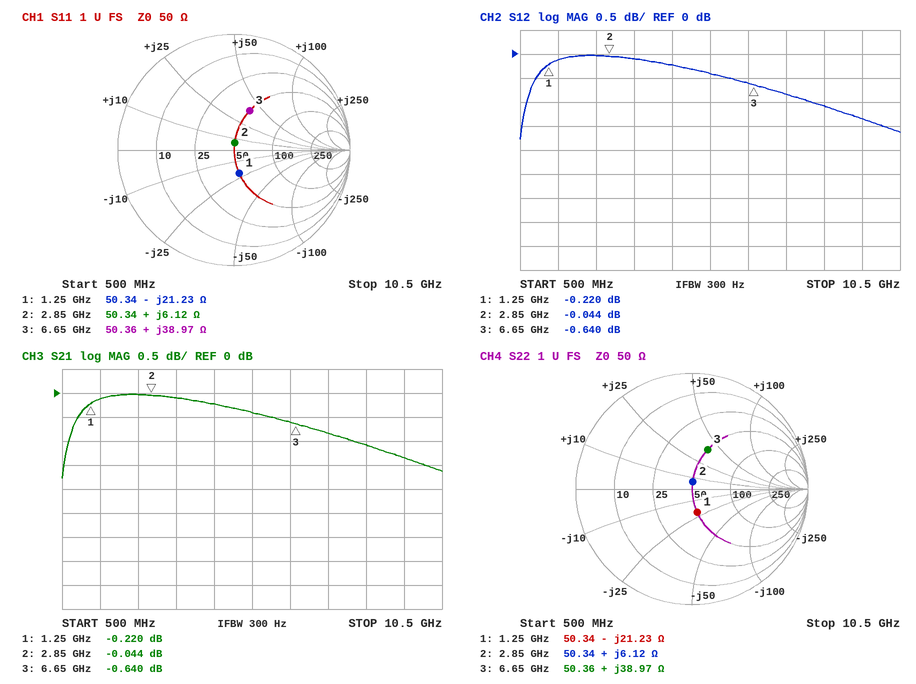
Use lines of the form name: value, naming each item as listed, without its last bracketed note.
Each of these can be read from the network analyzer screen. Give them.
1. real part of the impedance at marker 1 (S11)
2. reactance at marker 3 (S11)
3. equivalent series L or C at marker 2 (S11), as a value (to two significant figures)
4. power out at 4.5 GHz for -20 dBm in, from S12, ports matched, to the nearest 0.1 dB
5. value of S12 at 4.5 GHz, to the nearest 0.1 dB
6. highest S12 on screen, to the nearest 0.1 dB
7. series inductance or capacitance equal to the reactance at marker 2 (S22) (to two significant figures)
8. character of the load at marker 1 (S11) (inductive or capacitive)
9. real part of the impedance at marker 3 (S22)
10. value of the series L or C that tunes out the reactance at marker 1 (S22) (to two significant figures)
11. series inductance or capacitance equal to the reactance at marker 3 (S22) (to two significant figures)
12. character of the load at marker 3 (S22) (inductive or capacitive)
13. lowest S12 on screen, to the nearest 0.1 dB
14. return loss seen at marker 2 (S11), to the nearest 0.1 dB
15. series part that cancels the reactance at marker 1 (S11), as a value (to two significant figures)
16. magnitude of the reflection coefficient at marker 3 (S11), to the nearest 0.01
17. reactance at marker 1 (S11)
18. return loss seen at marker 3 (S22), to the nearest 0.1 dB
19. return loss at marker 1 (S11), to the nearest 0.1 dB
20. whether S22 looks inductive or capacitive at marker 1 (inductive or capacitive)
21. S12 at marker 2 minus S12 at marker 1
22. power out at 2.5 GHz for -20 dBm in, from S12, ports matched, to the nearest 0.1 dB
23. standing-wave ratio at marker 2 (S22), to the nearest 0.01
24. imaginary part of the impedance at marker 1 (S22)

real part of the impedance at marker 1: 50.34 Ω
reactance at marker 3: +38.97 Ω
equivalent series L or C at marker 2 (S11), as a value: 340 pH
power out at 4.5 GHz for -20 dBm in, from S12, ports matched, to the nearest 0.1 dB: -20.2 dBm
value of S12 at 4.5 GHz, to the nearest 0.1 dB: -0.2 dB
highest S12 on screen, to the nearest 0.1 dB: 0.0 dB
series inductance or capacitance equal to the reactance at marker 2 (S22): 340 pH
character of the load at marker 1 (S11): capacitive
real part of the impedance at marker 3: 50.36 Ω
value of the series L or C that tunes out the reactance at marker 1 (S22): 2.7 nH
series inductance or capacitance equal to the reactance at marker 3 (S22): 930 pH
character of the load at marker 3 (S22): inductive
lowest S12 on screen, to the nearest 0.1 dB: -1.8 dB
return loss seen at marker 2 (S11), to the nearest 0.1 dB: 24.3 dB
series part that cancels the reactance at marker 1 (S11), as a value: 2.7 nH
magnitude of the reflection coefficient at marker 3 (S11), to the nearest 0.01: 0.36
reactance at marker 1: -21.23 Ω
return loss seen at marker 3 (S22), to the nearest 0.1 dB: 8.8 dB
return loss at marker 1 (S11), to the nearest 0.1 dB: 13.7 dB
whether S22 looks inductive or capacitive at marker 1: capacitive
S12 at marker 2 minus S12 at marker 1: 0.176 dB
power out at 2.5 GHz for -20 dBm in, from S12, ports matched, to the nearest 0.1 dB: -20.0 dBm
standing-wave ratio at marker 2 (S22), to the nearest 0.01: 1.13
imaginary part of the impedance at marker 1: -21.23 Ω
